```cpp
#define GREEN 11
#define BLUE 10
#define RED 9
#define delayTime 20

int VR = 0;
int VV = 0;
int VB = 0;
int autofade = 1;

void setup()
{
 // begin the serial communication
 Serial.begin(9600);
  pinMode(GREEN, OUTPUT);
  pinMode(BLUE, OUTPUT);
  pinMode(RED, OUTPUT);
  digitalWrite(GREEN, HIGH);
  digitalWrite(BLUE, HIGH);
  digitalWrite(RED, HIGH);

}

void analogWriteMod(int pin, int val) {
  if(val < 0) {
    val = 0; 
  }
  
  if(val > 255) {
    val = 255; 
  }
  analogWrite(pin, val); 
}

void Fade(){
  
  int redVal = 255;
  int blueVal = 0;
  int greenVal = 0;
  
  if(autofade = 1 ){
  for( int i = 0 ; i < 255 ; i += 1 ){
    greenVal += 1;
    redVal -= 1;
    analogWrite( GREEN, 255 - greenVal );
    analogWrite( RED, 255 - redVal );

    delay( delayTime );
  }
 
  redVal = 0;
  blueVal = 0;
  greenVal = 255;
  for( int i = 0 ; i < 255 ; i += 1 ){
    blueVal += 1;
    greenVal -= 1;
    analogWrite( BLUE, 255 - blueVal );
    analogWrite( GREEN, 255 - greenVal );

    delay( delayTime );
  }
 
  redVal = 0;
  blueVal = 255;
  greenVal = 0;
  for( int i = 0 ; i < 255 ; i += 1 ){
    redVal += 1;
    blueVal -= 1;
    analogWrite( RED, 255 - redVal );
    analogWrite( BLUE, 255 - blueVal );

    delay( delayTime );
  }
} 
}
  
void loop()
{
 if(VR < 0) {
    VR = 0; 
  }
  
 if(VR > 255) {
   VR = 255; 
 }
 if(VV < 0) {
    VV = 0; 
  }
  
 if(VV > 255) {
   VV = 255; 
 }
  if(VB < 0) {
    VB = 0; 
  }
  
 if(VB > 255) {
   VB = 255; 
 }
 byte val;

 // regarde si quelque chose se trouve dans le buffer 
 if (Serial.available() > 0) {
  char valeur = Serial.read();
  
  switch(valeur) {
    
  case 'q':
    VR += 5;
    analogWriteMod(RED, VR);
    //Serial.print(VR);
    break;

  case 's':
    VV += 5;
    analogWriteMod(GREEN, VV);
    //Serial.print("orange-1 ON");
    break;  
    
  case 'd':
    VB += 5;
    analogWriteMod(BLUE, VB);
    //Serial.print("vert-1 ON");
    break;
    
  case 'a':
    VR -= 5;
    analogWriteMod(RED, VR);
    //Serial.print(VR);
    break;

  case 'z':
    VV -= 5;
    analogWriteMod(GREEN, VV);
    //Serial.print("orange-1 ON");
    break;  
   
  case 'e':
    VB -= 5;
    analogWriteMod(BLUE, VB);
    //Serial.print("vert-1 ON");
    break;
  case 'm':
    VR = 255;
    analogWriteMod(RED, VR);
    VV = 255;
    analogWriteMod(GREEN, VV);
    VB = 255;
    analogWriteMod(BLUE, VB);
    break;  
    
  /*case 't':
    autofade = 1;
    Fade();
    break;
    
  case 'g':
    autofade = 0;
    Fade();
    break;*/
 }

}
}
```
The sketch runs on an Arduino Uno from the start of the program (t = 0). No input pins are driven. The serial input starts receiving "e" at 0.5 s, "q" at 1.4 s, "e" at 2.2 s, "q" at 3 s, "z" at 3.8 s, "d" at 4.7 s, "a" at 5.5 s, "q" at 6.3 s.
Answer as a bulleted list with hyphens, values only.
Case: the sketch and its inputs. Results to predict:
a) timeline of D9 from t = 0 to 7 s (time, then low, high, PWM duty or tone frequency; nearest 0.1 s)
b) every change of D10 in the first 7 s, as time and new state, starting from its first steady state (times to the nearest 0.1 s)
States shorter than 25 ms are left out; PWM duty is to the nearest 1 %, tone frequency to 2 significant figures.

- 0 s high; 1.4 s PWM 2 %; 3 s PWM 4 %; 5.5 s PWM 2 %; 6.3 s PWM 4 %
- 0 s high; 0.5 s low; 4.7 s PWM 2 %
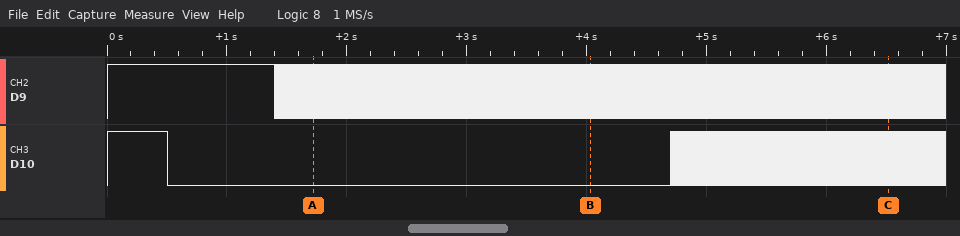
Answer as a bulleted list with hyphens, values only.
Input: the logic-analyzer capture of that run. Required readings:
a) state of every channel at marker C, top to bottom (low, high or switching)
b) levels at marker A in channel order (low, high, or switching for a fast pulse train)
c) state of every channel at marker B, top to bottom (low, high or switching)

- D9 switching, D10 switching
- D9 switching, D10 low
- D9 switching, D10 low
